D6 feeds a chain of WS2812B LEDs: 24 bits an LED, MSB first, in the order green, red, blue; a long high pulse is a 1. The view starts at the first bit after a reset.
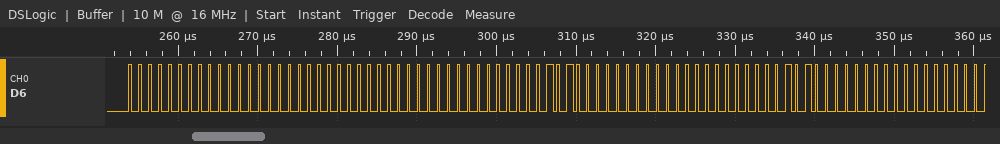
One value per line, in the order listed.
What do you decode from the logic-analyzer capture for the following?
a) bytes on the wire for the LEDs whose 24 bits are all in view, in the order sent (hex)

00 00 00 00 00 28 00 00 28
